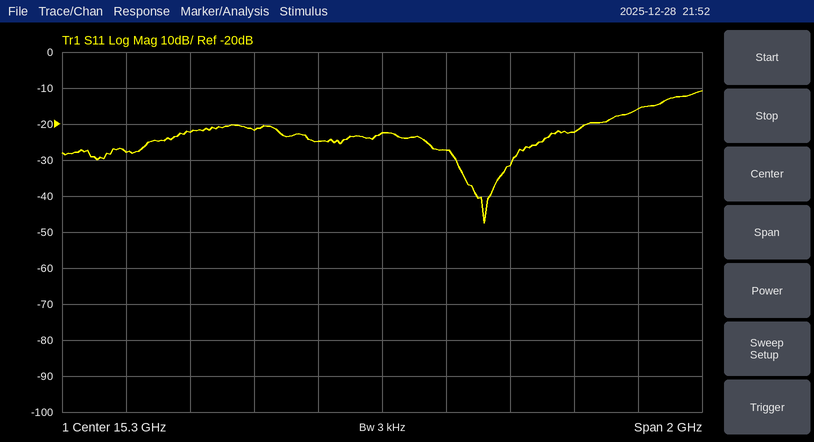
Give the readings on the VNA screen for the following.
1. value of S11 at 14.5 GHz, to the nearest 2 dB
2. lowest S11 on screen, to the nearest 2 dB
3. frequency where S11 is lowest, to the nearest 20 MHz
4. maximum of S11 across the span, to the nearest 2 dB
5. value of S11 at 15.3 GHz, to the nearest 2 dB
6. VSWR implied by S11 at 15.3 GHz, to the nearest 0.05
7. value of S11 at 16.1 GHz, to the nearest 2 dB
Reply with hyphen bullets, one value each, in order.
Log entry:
- -28 dB
- -48 dB
- 15.62 GHz
- -10 dB
- -22 dB
- 1.15
- -16 dB
